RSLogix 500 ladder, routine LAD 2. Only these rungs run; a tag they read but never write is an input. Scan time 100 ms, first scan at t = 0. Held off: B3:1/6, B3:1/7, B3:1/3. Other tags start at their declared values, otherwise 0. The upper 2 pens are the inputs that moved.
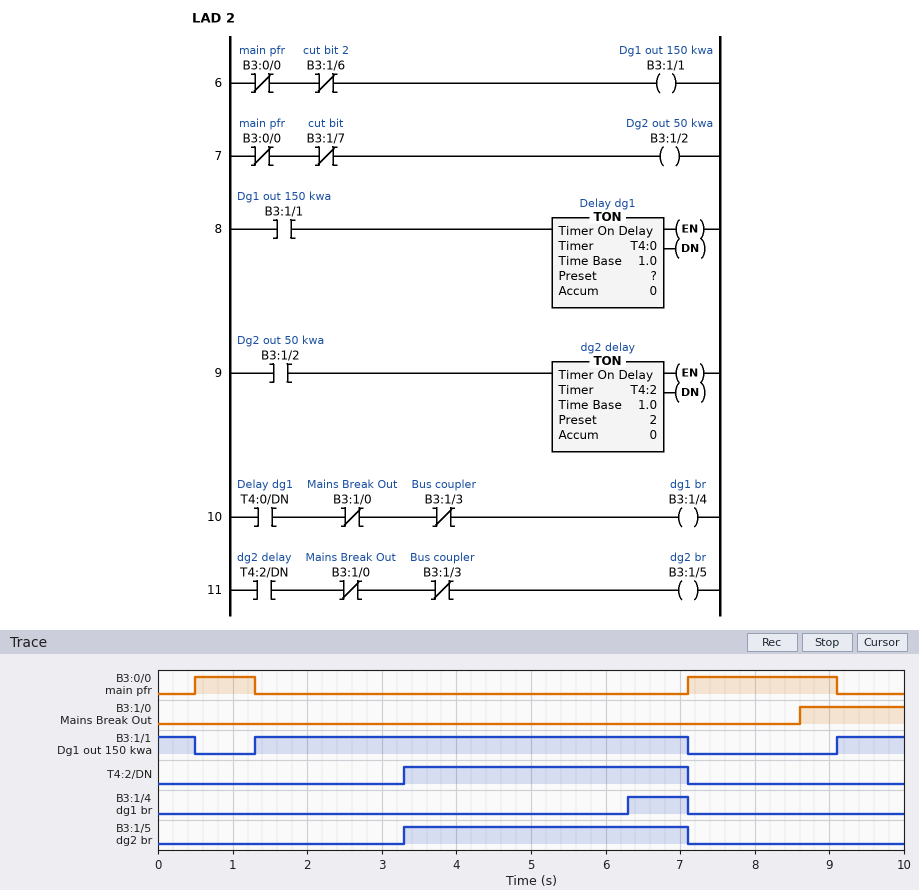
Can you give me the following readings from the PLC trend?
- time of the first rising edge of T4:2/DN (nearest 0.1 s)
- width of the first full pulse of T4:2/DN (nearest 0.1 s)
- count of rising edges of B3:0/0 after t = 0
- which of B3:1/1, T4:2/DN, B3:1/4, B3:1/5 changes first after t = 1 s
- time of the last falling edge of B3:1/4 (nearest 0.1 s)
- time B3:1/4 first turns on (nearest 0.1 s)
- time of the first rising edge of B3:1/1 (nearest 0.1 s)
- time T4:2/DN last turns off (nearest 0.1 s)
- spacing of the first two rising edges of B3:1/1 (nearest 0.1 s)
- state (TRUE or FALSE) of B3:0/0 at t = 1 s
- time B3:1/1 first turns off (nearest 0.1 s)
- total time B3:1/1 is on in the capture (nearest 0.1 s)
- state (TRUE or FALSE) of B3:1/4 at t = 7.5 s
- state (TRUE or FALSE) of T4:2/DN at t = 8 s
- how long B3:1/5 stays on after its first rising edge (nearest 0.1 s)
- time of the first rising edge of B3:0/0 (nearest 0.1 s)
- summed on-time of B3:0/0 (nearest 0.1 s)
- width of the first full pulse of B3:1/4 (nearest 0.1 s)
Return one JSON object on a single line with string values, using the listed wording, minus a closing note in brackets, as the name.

{"time of the first rising edge of T4:2/DN": "3.3 s", "width of the first full pulse of T4:2/DN": "3.8 s", "count of rising edges of B3:0/0 after t = 0": "2", "which of B3:1/1, T4:2/DN, B3:1/4, B3:1/5 changes first after t = 1 s": "B3:1/1", "time of the last falling edge of B3:1/4": "7.1 s", "time B3:1/4 first turns on": "6.3 s", "time of the first rising edge of B3:1/1": "1.3 s", "time T4:2/DN last turns off": "7.1 s", "spacing of the first two rising edges of B3:1/1": "7.8 s", "state (TRUE or FALSE) of B3:0/0 at t = 1 s": "TRUE", "time B3:1/1 first turns off": "0.5 s", "total time B3:1/1 is on in the capture": "7.2 s", "state (TRUE or FALSE) of B3:1/4 at t = 7.5 s": "FALSE", "state (TRUE or FALSE) of T4:2/DN at t = 8 s": "FALSE", "how long B3:1/5 stays on after its first rising edge": "3.8 s", "time of the first rising edge of B3:0/0": "0.5 s", "summed on-time of B3:0/0": "2.8 s", "width of the first full pulse of B3:1/4": "0.8 s"}
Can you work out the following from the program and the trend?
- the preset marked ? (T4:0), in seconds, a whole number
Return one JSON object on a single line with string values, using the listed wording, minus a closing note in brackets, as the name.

{"the preset marked ? (T4:0), in seconds, a whole number": "5 s"}
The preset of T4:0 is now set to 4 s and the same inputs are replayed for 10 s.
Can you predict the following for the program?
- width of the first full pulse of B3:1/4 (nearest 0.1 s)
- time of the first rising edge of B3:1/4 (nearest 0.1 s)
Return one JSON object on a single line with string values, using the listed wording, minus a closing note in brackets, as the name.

{"width of the first full pulse of B3:1/4": "1.8 s", "time of the first rising edge of B3:1/4": "5.3 s"}
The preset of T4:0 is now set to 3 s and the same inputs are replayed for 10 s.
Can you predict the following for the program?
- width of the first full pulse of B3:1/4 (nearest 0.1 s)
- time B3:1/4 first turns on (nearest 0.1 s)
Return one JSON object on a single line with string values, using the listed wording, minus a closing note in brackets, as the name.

{"width of the first full pulse of B3:1/4": "2.8 s", "time B3:1/4 first turns on": "4.3 s"}
